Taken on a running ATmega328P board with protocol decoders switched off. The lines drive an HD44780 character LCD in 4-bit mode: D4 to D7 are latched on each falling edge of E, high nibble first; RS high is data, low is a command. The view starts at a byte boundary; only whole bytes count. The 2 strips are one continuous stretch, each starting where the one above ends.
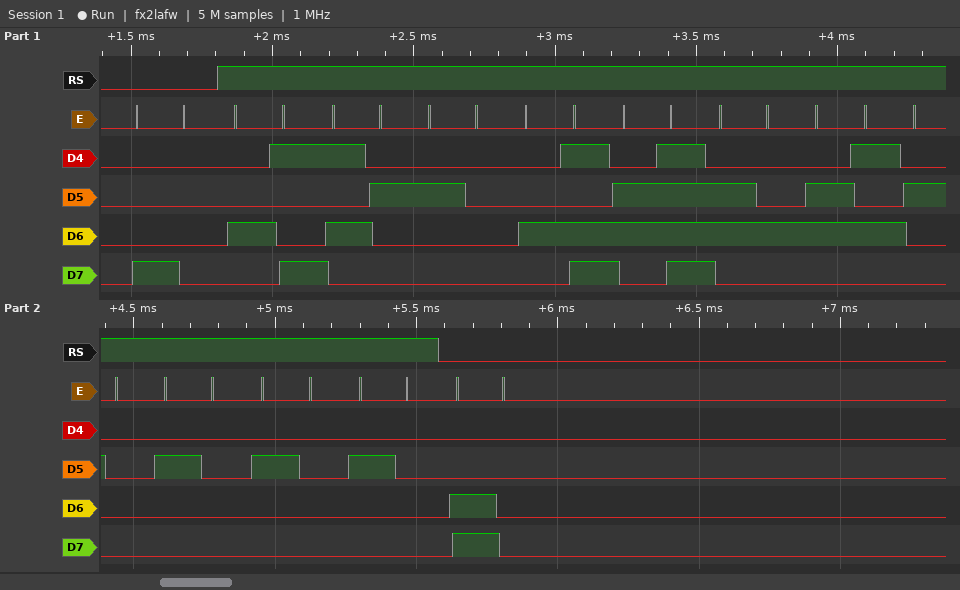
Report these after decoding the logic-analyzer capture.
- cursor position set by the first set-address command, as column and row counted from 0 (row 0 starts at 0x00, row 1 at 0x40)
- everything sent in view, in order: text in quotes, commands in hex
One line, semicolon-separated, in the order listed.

column 0, row 0; 0x80 "IR Mode    " 0xC0
